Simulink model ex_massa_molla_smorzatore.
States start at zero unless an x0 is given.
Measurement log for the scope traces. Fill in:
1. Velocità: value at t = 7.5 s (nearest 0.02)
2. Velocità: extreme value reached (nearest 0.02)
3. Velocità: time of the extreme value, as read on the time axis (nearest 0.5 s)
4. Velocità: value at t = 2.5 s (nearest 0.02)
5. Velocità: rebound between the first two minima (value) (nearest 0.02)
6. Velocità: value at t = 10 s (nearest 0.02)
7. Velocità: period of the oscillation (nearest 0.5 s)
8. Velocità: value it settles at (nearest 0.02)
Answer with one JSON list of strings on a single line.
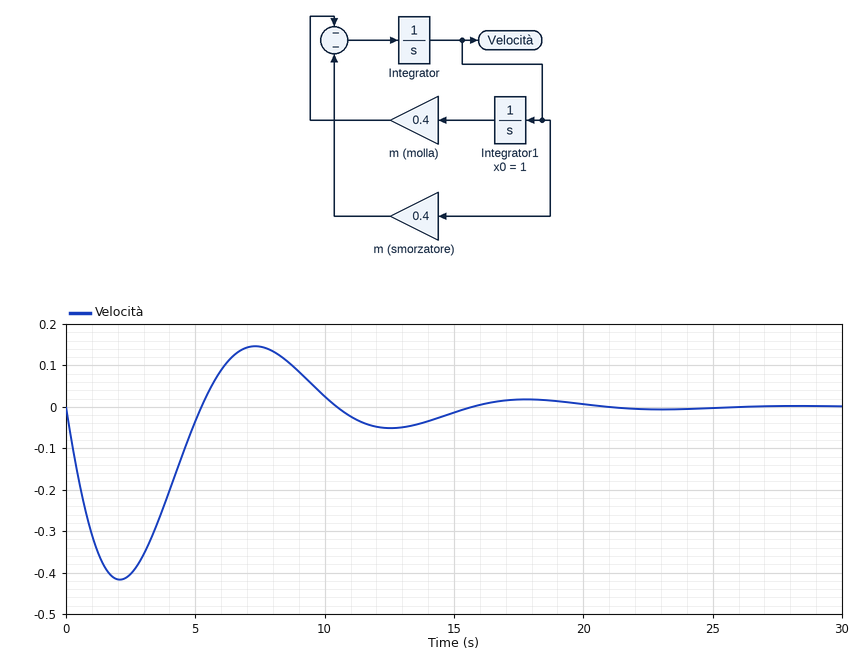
["0.14", "-0.42", "2.0 s", "-0.40", "0.14", "0.02", "10.5 s", "0.00"]
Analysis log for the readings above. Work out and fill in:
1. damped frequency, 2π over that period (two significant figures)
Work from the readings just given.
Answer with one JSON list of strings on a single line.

["0.60 rad/s"]
